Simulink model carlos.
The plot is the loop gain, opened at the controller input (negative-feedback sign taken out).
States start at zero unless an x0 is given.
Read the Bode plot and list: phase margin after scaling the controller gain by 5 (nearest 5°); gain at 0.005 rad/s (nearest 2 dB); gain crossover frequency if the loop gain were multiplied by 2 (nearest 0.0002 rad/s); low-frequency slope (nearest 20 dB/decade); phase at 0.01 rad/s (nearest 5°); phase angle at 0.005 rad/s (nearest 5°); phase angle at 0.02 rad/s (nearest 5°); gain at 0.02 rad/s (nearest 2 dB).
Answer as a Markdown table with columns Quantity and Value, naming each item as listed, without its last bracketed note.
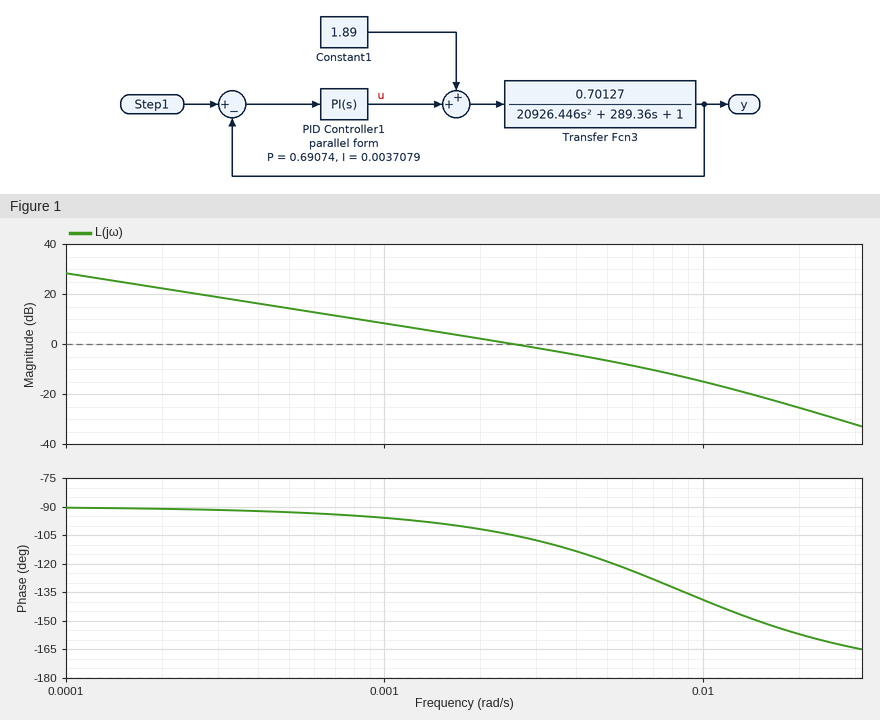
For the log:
| Quantity | Value |
|---|---|
| phase margin after scaling the controller gain by 5 | 45° |
| gain at 0.005 rad/s | -6 dB |
| gain crossover frequency if the loop gain were multiplied by 2 | 0.0048 rad/s |
| low-frequency slope | -20 dB/decade |
| phase at 0.01 rad/s | -140° |
| phase angle at 0.005 rad/s | -120° |
| phase angle at 0.02 rad/s | -155° |
| gain at 0.02 rad/s | -26 dB |
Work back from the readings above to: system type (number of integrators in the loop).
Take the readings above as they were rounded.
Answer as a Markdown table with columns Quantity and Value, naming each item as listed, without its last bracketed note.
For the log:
| Quantity | Value |
|---|---|
| system type | 1 |
